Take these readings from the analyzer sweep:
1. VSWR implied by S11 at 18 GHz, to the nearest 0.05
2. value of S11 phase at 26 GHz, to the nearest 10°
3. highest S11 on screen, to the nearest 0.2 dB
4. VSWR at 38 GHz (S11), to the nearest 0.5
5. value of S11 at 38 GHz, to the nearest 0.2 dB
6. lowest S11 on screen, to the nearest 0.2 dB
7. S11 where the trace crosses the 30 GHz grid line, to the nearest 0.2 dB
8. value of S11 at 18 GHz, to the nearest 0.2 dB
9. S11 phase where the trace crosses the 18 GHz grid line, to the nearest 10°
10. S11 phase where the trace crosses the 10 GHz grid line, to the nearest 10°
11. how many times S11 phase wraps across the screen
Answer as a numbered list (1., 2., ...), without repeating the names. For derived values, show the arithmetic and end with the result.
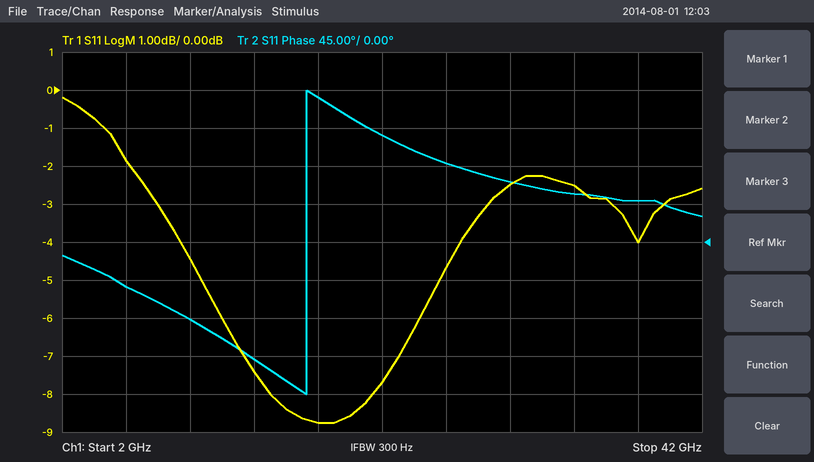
1. |Γ| = 10^(-8.8/20) = 0.3631; VSWR = (1 + 0.3631)/(1 − 0.3631) ≈ 2.14, so 2.15 to the nearest 0.05
2. 90°
3. -0.2 dB
4. |Γ| = 10^(-4/20) = 0.6310; VSWR = (1 + 0.6310)/(1 − 0.6310) ≈ 4.42, so 4.5 to the nearest 0.5
5. -4.0 dB
6. -8.8 dB
7. -2.4 dB
8. -8.8 dB
9. 170°
10. -90°
11. 1
